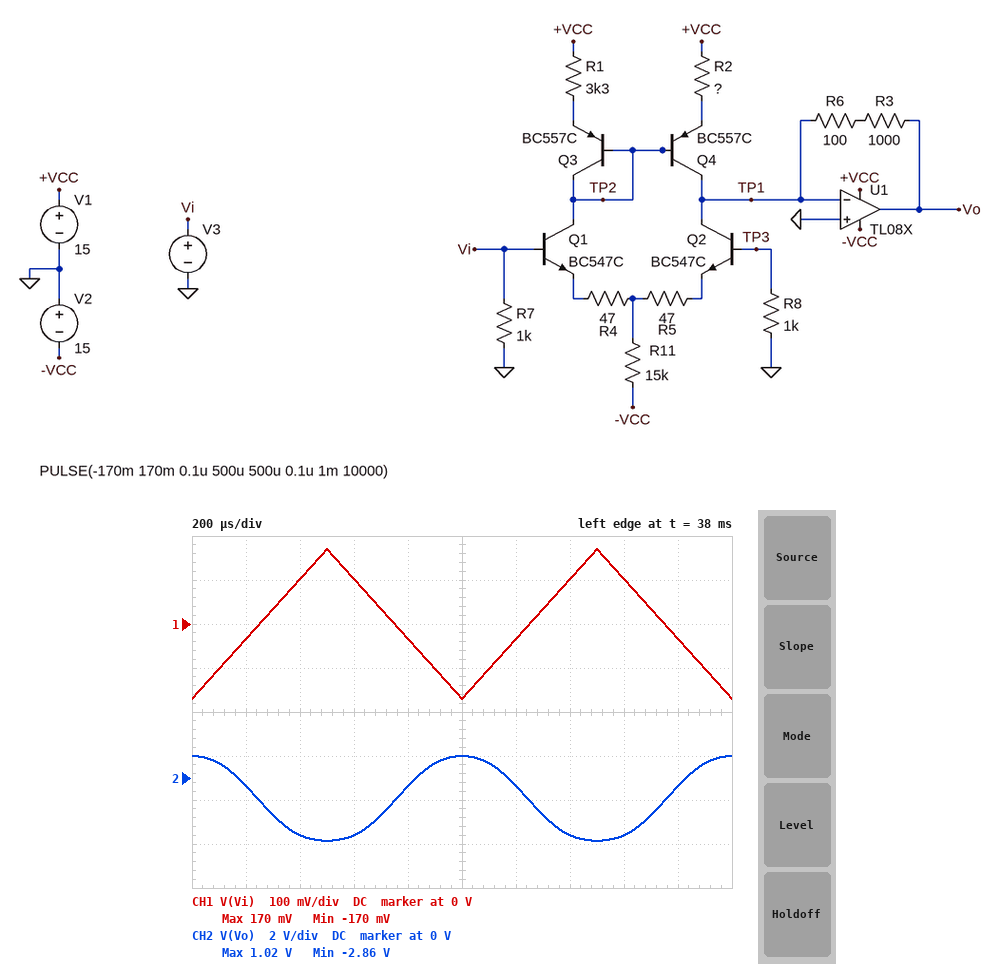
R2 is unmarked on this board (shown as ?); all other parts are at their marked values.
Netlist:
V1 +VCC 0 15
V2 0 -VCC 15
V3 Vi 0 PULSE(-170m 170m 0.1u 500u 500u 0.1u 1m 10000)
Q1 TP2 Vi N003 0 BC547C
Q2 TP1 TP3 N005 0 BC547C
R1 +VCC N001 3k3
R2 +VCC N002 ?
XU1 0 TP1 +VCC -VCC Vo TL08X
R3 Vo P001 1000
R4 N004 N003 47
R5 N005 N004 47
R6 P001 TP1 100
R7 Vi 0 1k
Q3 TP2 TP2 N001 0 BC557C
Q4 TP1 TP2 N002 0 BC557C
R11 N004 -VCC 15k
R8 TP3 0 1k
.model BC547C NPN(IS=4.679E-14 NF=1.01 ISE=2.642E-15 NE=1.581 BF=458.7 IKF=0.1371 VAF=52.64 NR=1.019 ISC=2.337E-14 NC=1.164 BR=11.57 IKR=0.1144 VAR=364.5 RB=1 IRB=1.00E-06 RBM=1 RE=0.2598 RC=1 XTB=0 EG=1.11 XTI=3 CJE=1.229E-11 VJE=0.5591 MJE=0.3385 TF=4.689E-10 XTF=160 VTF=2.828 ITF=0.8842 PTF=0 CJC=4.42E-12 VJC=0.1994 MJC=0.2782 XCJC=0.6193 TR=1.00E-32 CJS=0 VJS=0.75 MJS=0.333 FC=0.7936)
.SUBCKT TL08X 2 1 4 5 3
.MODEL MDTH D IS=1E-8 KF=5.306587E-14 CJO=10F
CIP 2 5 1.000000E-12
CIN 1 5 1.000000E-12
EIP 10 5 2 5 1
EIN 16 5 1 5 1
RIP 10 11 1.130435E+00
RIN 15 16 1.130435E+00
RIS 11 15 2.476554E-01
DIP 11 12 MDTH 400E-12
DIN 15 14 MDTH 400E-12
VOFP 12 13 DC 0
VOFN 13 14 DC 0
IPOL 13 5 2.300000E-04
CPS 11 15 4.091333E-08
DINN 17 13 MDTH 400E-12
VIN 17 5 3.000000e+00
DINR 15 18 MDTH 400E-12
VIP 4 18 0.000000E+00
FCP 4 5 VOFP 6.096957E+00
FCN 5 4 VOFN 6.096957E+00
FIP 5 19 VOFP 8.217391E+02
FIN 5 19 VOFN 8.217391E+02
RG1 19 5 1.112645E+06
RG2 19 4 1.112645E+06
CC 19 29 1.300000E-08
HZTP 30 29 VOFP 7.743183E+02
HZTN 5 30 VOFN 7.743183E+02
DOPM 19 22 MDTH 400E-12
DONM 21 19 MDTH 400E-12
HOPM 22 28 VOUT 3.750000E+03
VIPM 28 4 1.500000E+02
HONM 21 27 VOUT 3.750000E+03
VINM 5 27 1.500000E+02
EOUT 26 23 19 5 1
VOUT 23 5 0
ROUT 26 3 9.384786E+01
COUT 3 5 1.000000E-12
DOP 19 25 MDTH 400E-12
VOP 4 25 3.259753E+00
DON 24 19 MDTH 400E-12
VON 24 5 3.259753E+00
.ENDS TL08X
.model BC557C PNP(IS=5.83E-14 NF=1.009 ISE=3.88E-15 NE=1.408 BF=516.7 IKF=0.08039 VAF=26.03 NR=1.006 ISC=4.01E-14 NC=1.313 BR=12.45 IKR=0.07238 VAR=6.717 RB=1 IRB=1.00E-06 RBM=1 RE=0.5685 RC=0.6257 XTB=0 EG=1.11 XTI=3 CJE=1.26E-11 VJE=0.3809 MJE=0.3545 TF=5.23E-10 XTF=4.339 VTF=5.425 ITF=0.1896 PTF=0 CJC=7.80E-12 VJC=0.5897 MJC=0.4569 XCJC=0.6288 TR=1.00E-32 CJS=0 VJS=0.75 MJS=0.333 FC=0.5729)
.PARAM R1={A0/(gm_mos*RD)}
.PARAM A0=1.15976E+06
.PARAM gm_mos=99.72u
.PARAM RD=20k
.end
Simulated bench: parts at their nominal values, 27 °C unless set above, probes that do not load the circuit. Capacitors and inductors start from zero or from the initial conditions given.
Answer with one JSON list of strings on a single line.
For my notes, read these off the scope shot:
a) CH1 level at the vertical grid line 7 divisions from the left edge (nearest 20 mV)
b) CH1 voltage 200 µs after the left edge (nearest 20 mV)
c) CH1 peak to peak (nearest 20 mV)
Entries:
["100 mV", "-40 mV", "340 mV"]
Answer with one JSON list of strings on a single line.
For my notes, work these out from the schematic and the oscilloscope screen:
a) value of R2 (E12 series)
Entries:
["1.2 kΩ"]
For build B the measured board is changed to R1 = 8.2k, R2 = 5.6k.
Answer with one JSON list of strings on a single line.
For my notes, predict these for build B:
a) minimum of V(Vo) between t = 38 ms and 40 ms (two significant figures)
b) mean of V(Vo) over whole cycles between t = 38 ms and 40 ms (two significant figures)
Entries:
["-1.5 V", "-290 mV"]
